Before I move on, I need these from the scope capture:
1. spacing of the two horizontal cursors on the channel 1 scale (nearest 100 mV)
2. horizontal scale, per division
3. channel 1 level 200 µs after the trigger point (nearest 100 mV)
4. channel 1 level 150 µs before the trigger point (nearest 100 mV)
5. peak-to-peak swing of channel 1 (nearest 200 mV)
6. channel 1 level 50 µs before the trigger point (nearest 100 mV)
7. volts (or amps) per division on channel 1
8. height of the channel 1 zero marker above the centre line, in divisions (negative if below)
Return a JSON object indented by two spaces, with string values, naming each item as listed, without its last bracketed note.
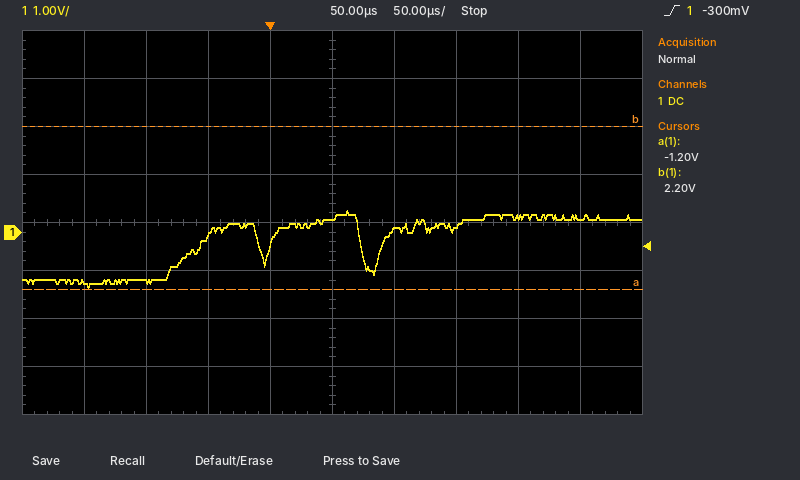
{
  "spacing of the two horizontal cursors on the channel 1 scale": "3.4 V",
  "horizontal scale, per division": "50 µs",
  "channel 1 level 200 µs after the trigger point": "300 mV",
  "channel 1 level 150 µs before the trigger point": "-1.0 V",
  "peak-to-peak swing of channel 1": "1.6 V",
  "channel 1 level 50 µs before the trigger point": "-100 mV",
  "volts (or amps) per division on channel 1": "1 V",
  "height of the channel 1 zero marker above the centre line, in divisions": "-0.2 div"
}
